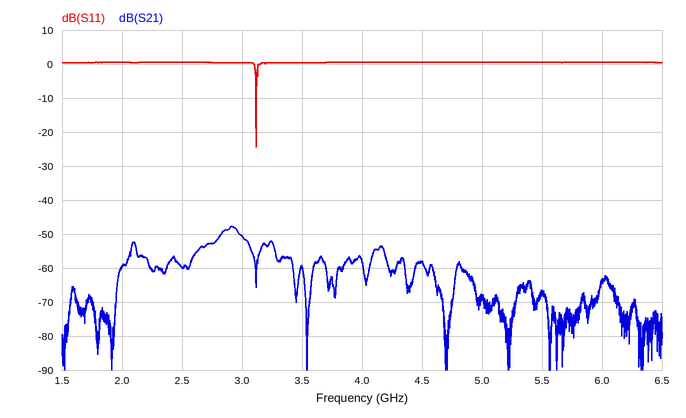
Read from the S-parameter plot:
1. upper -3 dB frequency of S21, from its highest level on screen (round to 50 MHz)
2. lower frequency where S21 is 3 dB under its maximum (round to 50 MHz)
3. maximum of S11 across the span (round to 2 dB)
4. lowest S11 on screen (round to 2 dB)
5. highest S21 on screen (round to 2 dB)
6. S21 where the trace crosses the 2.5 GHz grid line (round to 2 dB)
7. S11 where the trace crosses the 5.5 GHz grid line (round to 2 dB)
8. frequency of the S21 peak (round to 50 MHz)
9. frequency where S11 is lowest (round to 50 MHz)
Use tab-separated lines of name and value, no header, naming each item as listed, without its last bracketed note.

upper -3 dB frequency of S21, from its highest level on screen	3.00 GHz
lower frequency where S21 is 3 dB under its maximum	2.80 GHz
maximum of S11 across the span	0 dB
lowest S11 on screen	-24 dB
highest S21 on screen	-48 dB
S21 where the trace crosses the 2.5 GHz grid line	-60 dB
S11 where the trace crosses the 5.5 GHz grid line	0 dB
frequency of the S21 peak	2.90 GHz
frequency where S11 is lowest	3.10 GHz
